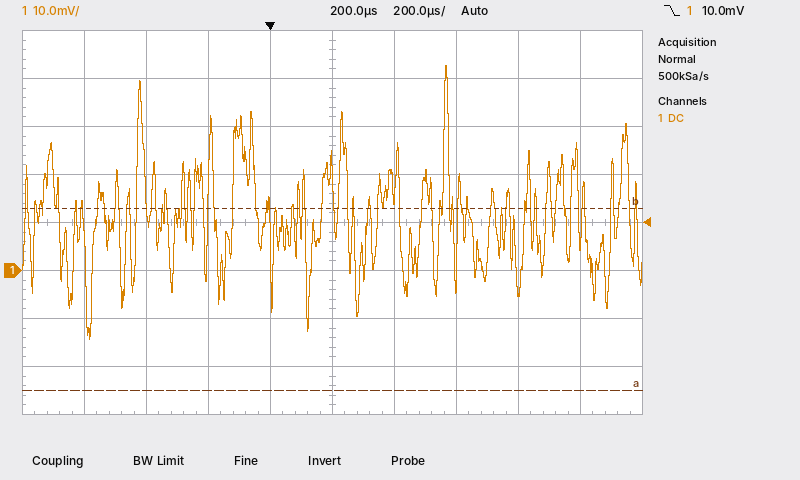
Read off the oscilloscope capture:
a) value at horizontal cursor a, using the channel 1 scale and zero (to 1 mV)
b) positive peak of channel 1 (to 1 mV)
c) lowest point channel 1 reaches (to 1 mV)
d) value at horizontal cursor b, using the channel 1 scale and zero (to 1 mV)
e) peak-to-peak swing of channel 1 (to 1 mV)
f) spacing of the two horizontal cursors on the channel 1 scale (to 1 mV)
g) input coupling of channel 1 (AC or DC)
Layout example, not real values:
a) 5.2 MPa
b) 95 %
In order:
a) -25 mV
b) 43 mV
c) -14 mV
d) 13 mV
e) 57 mV
f) 38 mV
g) DC
